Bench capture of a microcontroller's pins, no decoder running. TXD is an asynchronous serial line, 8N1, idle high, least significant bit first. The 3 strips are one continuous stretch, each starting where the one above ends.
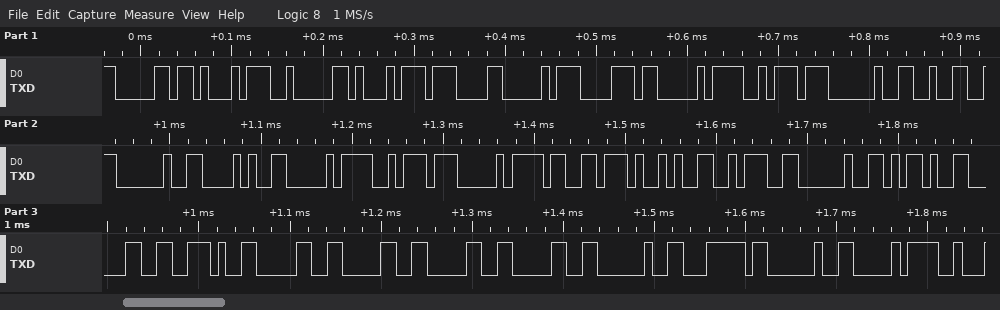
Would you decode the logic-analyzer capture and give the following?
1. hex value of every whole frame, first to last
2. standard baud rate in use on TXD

B0 D1 82 D1 87 D0 B8 D0 BA 20 32 20 28 D0 BA D0 B3 29 3A 20 2D 30 2E 30 30 30 30 20 7C 20 D0
115200 baud
